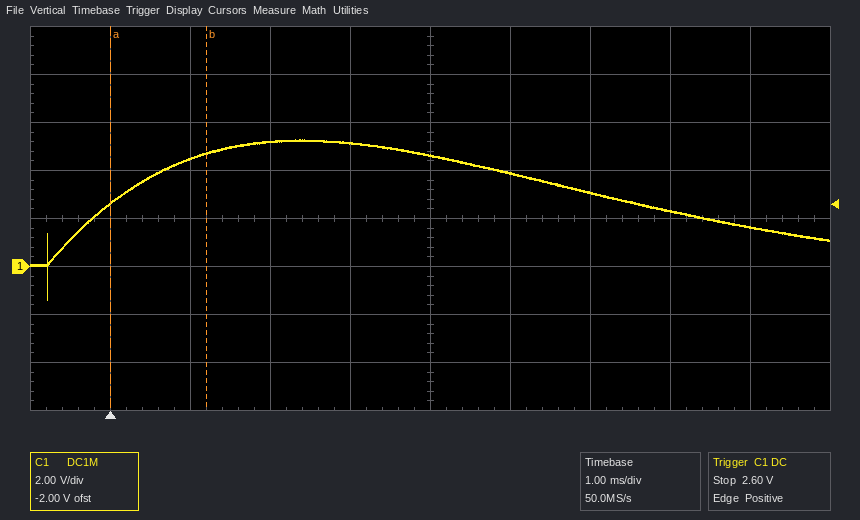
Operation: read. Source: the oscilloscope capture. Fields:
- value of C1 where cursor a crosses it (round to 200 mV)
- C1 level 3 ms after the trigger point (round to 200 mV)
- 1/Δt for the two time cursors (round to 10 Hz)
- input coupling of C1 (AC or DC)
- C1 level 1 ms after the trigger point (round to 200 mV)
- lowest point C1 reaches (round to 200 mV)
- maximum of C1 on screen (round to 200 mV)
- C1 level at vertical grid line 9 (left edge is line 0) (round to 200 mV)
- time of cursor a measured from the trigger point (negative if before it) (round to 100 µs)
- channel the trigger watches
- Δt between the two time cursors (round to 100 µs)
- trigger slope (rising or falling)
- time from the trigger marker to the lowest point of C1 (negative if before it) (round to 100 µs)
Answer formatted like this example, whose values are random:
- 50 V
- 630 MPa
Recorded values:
- 2.6 V
- 5.2 V
- 830 Hz
- DC
- 4.4 V
- -1.4 V
- 5.2 V
- 1.6 V
- 0.0 ms
- C1
- 1.2 ms
- rising
- -800 µs
